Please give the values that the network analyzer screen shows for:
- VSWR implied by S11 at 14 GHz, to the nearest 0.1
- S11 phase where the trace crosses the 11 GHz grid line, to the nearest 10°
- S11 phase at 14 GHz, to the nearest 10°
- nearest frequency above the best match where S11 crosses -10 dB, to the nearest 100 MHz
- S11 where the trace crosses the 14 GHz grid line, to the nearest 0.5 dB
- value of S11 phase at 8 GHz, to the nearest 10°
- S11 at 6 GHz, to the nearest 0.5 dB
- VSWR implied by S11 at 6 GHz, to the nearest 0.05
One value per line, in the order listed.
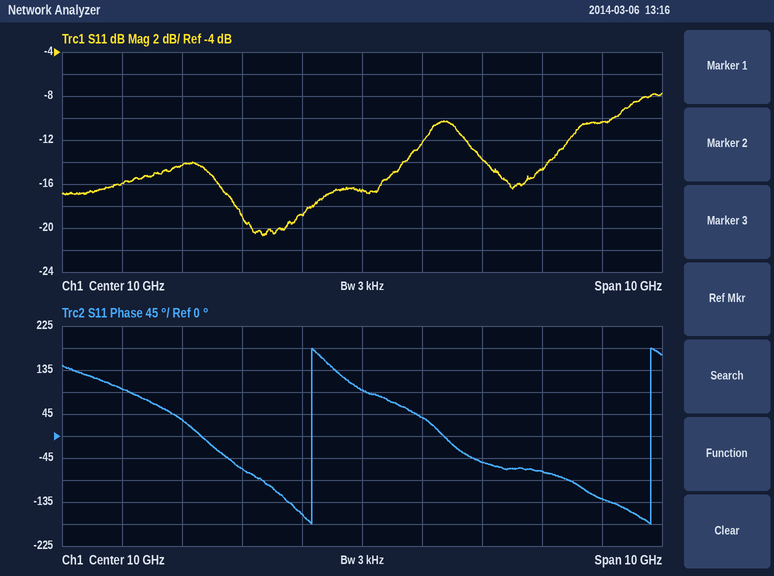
1.9
40°
-130°
14.2 GHz
-10.5 dB
-70°
-16.0 dB
1.40
